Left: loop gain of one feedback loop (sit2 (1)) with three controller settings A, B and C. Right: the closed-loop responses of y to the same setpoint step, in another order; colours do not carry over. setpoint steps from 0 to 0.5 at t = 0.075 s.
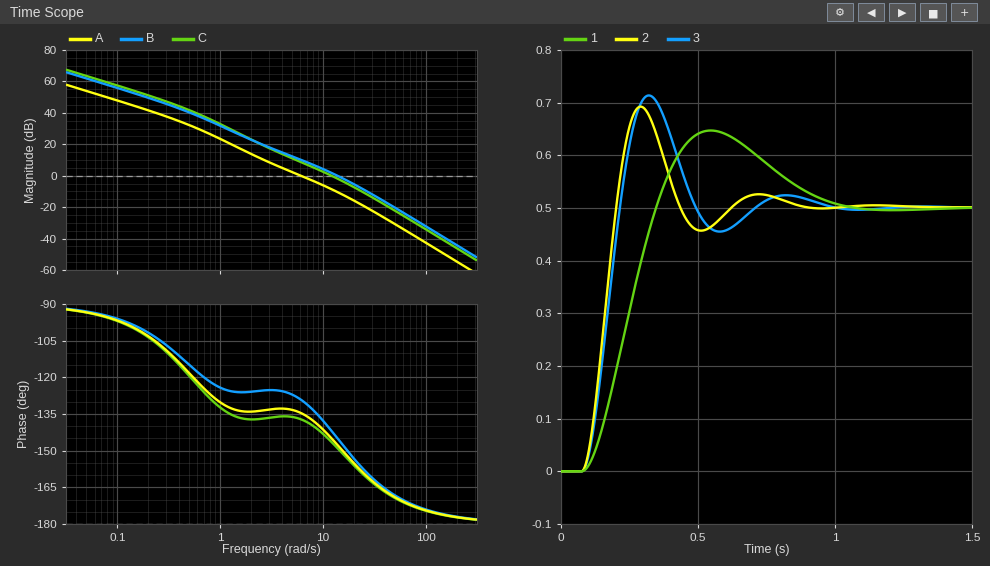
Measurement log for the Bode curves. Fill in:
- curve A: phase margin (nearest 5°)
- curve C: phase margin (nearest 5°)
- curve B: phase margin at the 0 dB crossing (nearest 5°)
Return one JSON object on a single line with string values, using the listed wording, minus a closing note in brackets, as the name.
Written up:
{"curve A: phase margin": "45°", "curve C: phase margin": "35°", "curve B: phase margin at the 0 dB crossing": "35°"}
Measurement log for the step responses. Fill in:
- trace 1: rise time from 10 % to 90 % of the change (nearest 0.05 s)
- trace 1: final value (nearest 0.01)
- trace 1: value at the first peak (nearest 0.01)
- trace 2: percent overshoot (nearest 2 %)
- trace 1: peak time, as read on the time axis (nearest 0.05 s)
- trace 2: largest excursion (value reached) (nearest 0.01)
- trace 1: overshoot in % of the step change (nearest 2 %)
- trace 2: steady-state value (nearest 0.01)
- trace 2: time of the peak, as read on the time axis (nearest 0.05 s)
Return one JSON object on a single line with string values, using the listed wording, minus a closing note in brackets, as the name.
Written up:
{"trace 1: rise time from 10 % to 90 % of the change": "0.20 s", "trace 1: final value": "0.50", "trace 1: value at the first peak": "0.65", "trace 2: percent overshoot": "38 %", "trace 1: peak time, as read on the time axis": "0.55 s", "trace 2: largest excursion (value reached)": "0.69", "trace 1: overshoot in % of the step change": "30 %", "trace 2: steady-state value": "0.50", "trace 2: time of the peak, as read on the time axis": "0.30 s"}
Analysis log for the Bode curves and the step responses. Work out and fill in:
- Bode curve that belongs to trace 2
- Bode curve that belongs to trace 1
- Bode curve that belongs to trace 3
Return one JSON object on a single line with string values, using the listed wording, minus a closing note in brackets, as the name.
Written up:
{"Bode curve that belongs to trace 2": "B", "Bode curve that belongs to trace 1": "A", "Bode curve that belongs to trace 3": "C"}
